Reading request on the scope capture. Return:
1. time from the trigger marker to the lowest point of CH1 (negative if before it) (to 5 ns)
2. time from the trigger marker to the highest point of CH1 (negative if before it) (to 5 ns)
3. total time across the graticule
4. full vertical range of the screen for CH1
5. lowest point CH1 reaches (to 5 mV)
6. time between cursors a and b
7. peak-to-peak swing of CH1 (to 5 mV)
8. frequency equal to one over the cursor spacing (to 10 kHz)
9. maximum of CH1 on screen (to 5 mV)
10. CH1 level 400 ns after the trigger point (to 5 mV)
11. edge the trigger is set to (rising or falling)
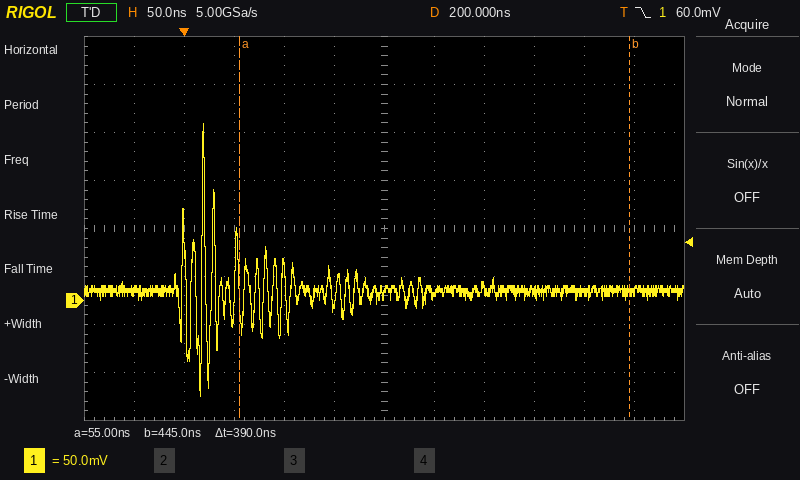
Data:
+15 ns
+20 ns
600 ns
400 mV
-100 mV
390 ns
285 mV
2.56 MHz
185 mV
10 mV
falling
